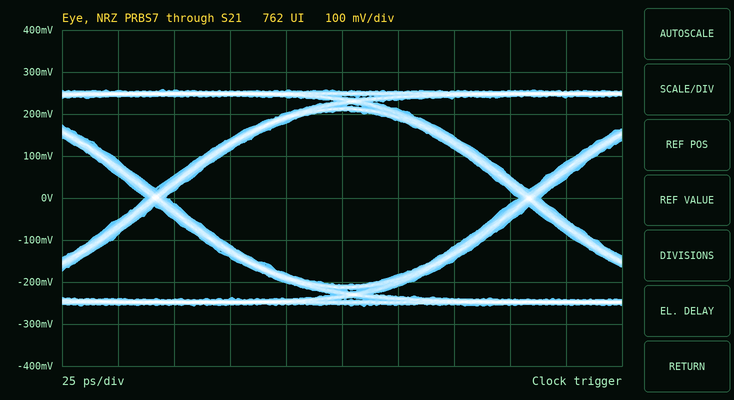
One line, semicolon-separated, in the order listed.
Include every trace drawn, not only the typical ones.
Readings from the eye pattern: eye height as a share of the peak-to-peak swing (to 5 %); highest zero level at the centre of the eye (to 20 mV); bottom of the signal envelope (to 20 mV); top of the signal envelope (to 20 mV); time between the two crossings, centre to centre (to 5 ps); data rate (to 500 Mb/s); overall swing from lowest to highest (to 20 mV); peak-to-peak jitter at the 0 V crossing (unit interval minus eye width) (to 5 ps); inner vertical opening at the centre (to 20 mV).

80 %; -200 mV; -260 mV; 260 mV; 165 ps; 6.0 Gb/s; 520 mV; 10 ps; 420 mV
